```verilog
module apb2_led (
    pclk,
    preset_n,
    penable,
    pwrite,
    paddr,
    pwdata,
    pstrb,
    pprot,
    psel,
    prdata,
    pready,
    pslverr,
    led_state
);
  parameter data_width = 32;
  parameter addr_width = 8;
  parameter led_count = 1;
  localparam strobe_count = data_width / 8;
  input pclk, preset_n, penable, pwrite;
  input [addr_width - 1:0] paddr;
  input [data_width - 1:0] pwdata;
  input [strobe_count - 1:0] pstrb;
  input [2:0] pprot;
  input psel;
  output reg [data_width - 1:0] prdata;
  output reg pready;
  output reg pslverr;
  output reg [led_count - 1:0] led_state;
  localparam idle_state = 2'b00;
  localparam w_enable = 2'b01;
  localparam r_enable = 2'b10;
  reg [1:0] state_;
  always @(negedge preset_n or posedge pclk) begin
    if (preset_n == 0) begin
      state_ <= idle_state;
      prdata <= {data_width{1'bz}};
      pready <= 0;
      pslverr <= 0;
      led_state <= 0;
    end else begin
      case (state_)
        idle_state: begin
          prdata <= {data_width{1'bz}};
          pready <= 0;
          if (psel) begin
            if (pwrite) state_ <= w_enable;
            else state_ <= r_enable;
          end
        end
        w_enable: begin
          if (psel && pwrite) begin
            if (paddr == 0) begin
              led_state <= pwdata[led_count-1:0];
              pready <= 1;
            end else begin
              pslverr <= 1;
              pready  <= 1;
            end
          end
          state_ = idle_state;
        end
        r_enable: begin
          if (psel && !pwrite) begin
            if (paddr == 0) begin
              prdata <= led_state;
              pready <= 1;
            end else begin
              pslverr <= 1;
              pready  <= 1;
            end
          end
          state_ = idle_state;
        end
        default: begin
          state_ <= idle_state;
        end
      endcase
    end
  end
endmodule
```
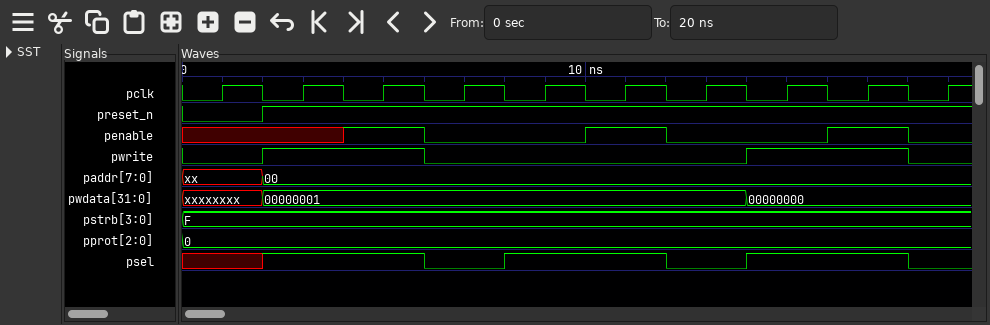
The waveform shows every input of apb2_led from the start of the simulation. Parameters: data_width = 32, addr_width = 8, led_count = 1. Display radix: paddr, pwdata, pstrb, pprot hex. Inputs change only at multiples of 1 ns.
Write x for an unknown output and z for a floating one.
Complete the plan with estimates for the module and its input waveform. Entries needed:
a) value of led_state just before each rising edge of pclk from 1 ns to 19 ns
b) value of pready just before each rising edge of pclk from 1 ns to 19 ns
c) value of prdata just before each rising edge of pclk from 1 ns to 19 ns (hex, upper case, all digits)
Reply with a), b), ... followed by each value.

a) 0 0 0 1 1 1 1 1 1 0
b) 0 0 0 1 0 0 1 0 0 1
c) z, z, z, z, z, z, 00000001, z, z, z
